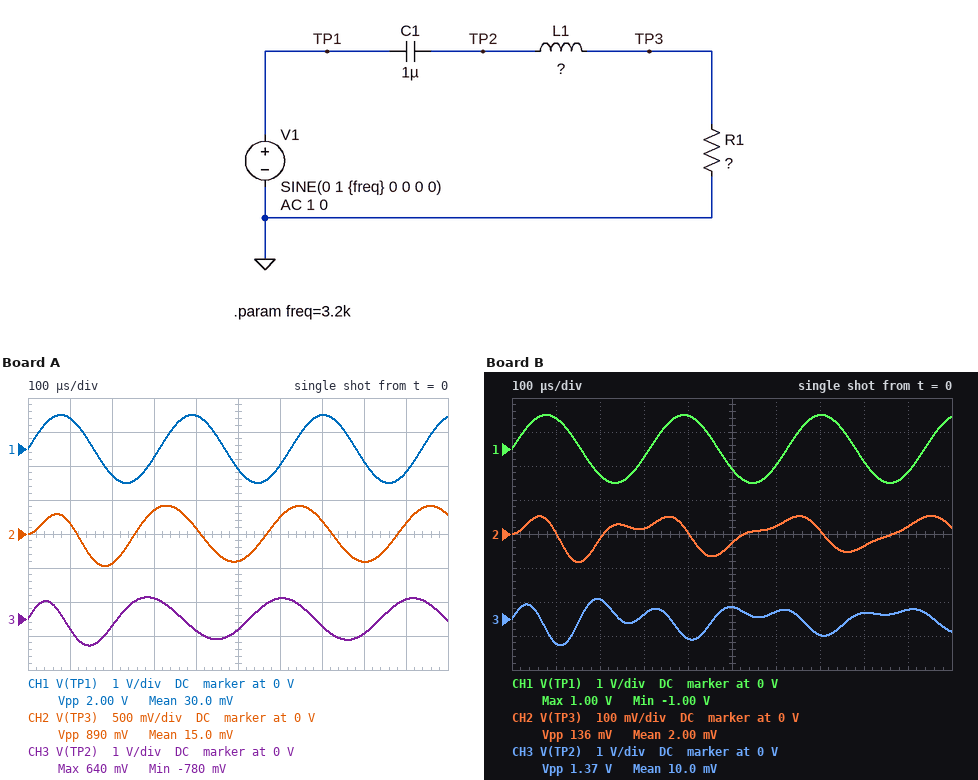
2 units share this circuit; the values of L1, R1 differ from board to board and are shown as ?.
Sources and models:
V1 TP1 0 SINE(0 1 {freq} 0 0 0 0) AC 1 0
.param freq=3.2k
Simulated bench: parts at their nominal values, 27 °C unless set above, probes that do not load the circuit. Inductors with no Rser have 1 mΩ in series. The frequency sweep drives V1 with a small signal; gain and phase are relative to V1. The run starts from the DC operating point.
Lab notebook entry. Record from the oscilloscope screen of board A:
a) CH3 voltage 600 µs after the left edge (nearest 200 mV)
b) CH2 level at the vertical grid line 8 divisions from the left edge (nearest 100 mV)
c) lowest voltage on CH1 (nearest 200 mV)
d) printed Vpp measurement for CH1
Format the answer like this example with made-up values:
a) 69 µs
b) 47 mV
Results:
a) 600 mV
b) -400 mV
c) -1.0 V
d) 2.00 V
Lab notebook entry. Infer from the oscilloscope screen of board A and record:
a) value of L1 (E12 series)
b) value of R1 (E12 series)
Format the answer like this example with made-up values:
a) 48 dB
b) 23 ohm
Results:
a) 820 µH
b) 15 Ω
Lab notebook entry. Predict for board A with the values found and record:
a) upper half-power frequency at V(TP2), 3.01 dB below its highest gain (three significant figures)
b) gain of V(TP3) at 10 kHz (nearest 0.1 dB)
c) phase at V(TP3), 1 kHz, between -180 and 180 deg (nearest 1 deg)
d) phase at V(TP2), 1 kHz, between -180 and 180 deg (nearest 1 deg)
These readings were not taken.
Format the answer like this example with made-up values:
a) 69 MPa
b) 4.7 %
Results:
a) 8.66 kHz
b) -8.2 dB
c) 84 deg
d) 103 deg
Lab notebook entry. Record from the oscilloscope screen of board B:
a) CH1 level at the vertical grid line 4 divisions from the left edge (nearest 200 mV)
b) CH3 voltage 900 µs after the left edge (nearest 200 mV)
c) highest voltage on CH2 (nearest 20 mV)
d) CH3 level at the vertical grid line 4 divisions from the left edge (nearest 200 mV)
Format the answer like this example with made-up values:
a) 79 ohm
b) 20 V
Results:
a) 1.0 V
b) 200 mV
c) 60 mV
d) -600 mV
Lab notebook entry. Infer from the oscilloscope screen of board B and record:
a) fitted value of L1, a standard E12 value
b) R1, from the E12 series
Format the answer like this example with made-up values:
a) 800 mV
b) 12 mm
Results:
a) 560 µH
b) 1.8 Ω
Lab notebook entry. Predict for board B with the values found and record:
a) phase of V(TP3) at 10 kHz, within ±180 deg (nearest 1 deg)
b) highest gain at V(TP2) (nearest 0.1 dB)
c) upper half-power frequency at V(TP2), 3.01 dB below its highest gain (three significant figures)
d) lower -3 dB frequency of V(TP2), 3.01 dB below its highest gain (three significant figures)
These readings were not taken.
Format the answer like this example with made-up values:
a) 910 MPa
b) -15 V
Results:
a) -85 deg
b) 22.4 dB
c) 7.01 kHz
d) 6.49 kHz
